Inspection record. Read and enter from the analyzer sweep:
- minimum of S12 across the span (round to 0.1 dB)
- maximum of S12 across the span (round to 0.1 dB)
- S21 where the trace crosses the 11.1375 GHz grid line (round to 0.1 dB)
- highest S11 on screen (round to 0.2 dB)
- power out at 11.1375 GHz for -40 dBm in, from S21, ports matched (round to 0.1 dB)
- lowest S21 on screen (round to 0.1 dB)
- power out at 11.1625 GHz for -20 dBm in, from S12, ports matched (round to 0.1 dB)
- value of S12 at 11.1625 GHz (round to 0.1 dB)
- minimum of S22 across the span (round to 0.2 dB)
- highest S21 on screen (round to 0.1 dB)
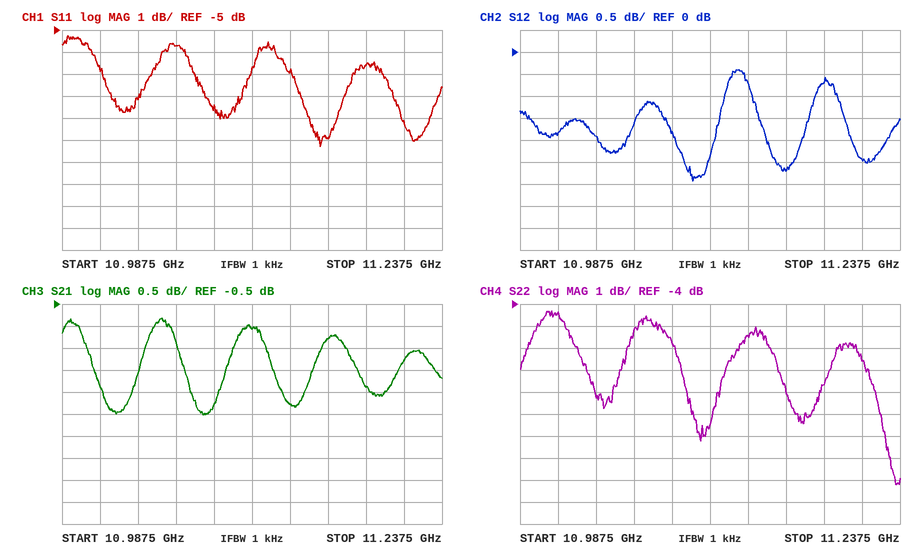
-2.9 dB
-0.4 dB
-2.8 dB
-5.2 dB
-42.8 dBm
-3.0 dB
-22.7 dBm
-2.7 dB
-12.2 dB
-0.8 dB
